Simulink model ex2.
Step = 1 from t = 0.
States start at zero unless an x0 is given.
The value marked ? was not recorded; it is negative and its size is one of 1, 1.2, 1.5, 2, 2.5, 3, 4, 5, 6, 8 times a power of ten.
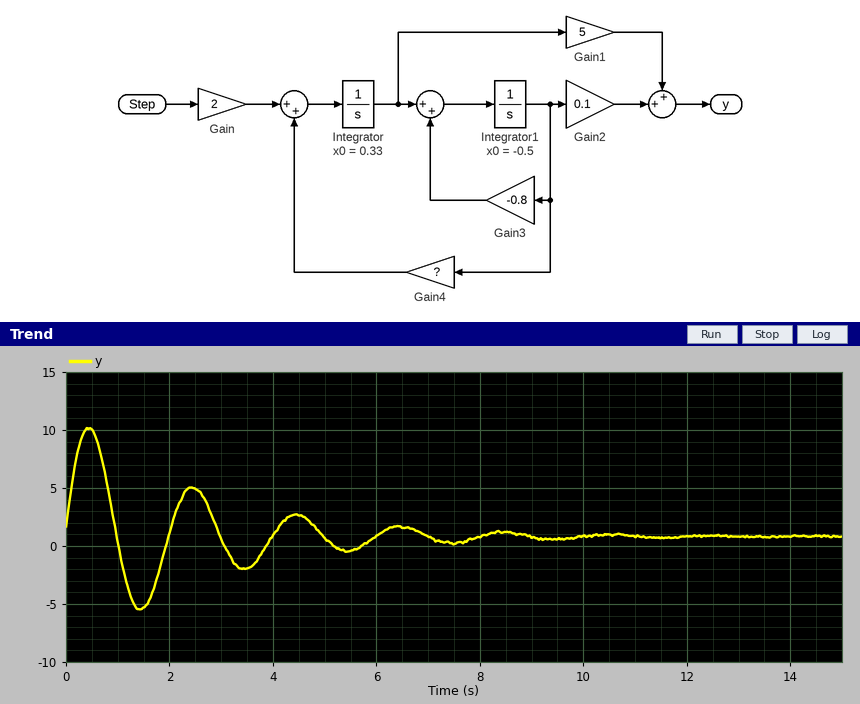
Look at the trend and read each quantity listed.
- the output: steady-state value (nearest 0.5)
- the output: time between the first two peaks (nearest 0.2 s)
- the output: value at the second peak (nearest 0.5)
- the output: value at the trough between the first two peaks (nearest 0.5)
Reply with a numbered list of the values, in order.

1. 1.0
2. 2.0 s
3. 5.0
4. -5.5
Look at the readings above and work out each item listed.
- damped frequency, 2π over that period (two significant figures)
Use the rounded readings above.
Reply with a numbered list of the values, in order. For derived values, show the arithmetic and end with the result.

1. 2π / 2 = 3.1 rad/s
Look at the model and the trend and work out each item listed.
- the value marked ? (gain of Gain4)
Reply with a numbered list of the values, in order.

1. -10
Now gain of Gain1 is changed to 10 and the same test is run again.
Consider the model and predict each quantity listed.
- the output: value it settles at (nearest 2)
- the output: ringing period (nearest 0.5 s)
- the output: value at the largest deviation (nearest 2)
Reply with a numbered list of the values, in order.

1. 2
2. 2.0 s
3. 20
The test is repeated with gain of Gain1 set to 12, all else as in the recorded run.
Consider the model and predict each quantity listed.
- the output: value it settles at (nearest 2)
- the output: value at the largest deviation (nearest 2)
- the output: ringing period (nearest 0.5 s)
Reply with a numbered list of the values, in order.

1. 2
2. 24
3. 2.0 s
